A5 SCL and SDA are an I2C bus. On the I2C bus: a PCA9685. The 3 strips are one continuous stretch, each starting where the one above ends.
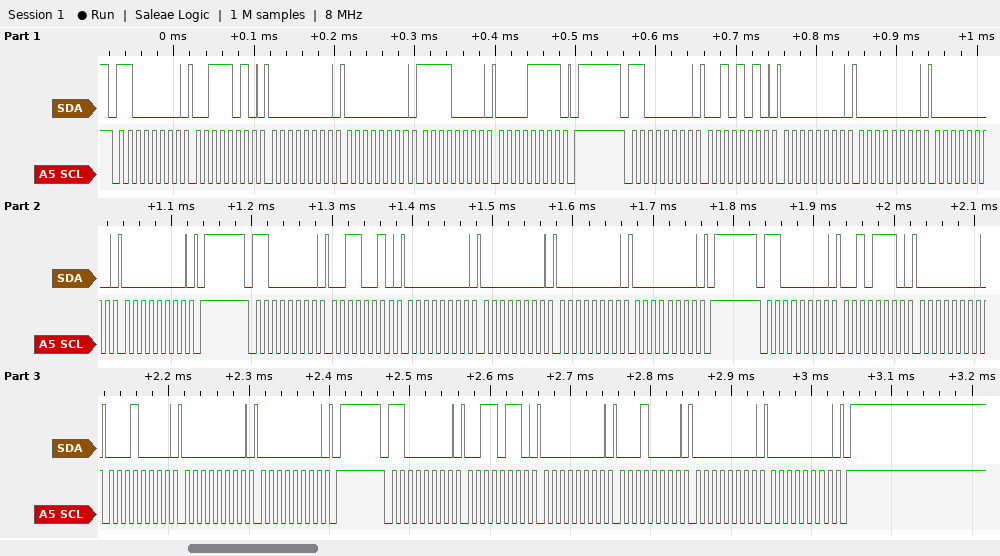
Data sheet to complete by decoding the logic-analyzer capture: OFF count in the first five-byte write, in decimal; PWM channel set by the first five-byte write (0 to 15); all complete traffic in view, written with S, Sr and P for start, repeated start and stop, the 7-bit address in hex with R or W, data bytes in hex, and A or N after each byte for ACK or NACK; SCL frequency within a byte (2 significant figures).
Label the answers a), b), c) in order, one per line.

a) 4080
b) 13
c) S 60W A 3A A 00 A 00 A F0 A 0F A P S 60W A 2A A 00 A 00 A 00 A 00 A P S 60W A 32 A 00 A 00 A 00 A 00 A P S 60W A 2E A 00 A 10 A 00 A 00 A P S 60W A 36 A 00 A 10 A 00 A 00 A P
d) 100 kHz
